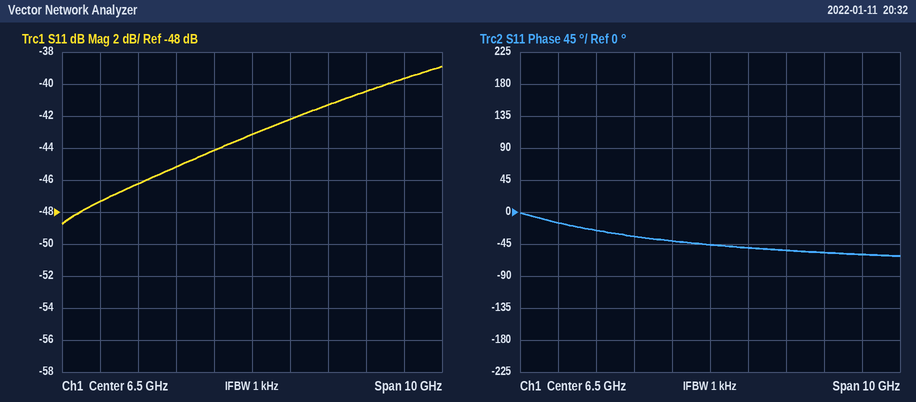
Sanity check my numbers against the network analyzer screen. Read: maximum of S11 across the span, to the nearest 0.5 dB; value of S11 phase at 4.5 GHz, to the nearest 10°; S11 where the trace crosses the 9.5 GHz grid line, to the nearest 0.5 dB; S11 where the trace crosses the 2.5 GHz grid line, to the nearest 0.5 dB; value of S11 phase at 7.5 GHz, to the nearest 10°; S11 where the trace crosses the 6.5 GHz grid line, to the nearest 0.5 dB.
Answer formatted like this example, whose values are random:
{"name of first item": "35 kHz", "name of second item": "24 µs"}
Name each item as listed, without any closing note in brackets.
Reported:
{"maximum of S11 across the span, to the nearest 0.5 dB": "-39.0 dB", "value of S11 phase at 4.5 GHz, to the nearest 10°": "-30°", "S11 where the trace crosses the 9.5 GHz grid line, to the nearest 0.5 dB": "-40.5 dB", "S11 where the trace crosses the 2.5 GHz grid line, to the nearest 0.5 dB": "-47.5 dB", "value of S11 phase at 7.5 GHz, to the nearest 10°": "-50°", "S11 where the trace crosses the 6.5 GHz grid line, to the nearest 0.5 dB": "-43.0 dB"}
